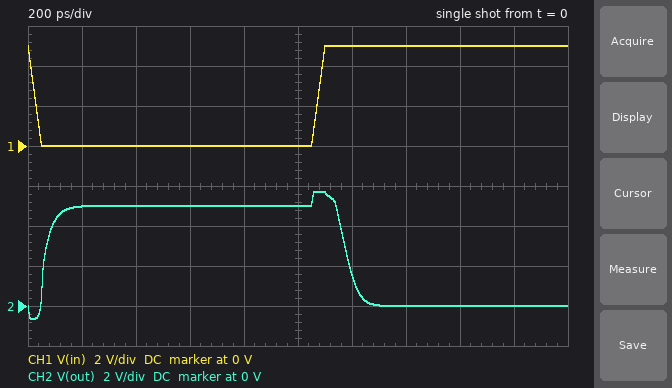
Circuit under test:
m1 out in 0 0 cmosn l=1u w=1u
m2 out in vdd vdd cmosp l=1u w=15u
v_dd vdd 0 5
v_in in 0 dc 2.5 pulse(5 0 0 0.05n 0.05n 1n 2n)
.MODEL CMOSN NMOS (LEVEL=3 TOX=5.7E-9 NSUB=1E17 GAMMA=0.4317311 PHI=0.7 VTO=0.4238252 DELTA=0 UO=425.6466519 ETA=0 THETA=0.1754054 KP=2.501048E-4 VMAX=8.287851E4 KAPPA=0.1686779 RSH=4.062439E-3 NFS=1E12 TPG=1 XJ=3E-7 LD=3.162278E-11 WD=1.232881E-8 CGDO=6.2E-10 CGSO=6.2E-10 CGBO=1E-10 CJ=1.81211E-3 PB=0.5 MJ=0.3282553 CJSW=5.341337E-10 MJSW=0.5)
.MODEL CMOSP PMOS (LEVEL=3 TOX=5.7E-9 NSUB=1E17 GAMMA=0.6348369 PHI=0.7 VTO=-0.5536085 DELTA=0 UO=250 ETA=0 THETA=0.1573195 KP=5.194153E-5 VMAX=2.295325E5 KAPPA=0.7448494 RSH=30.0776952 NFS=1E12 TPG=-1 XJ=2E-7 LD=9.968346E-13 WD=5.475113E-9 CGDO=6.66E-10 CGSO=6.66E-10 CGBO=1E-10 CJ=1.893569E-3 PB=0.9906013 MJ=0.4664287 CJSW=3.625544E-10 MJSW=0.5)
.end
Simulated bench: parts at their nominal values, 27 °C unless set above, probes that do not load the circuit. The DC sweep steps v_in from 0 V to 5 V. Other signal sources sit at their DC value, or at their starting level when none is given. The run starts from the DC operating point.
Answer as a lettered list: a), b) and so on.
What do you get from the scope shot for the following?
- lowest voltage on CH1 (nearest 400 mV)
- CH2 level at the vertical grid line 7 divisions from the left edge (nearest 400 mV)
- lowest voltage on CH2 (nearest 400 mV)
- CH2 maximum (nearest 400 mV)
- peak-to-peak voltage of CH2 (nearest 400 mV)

a) 0 V
b) 0 V
c) -800 mV
d) 5.6 V
e) 6.4 V
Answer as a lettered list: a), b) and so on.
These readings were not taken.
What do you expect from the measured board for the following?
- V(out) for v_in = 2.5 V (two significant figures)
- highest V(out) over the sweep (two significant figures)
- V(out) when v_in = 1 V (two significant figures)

a) 4.8 V
b) 5.0 V
c) 5.0 V
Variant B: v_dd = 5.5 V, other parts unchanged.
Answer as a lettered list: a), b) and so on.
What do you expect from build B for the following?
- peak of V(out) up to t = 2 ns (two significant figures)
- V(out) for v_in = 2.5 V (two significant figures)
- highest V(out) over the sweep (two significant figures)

a) 6.2 V
b) 5.3 V
c) 5.5 V
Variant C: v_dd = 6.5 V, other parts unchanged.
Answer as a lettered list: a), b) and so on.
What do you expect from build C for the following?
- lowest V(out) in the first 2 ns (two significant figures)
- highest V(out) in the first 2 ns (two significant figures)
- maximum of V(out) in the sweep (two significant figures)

a) -330 mV
b) 7.2 V
c) 6.5 V
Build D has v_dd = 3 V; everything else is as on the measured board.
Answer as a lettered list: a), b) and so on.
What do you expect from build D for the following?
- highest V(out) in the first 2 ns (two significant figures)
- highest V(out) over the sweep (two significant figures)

a) 3.7 V
b) 3.0 V
